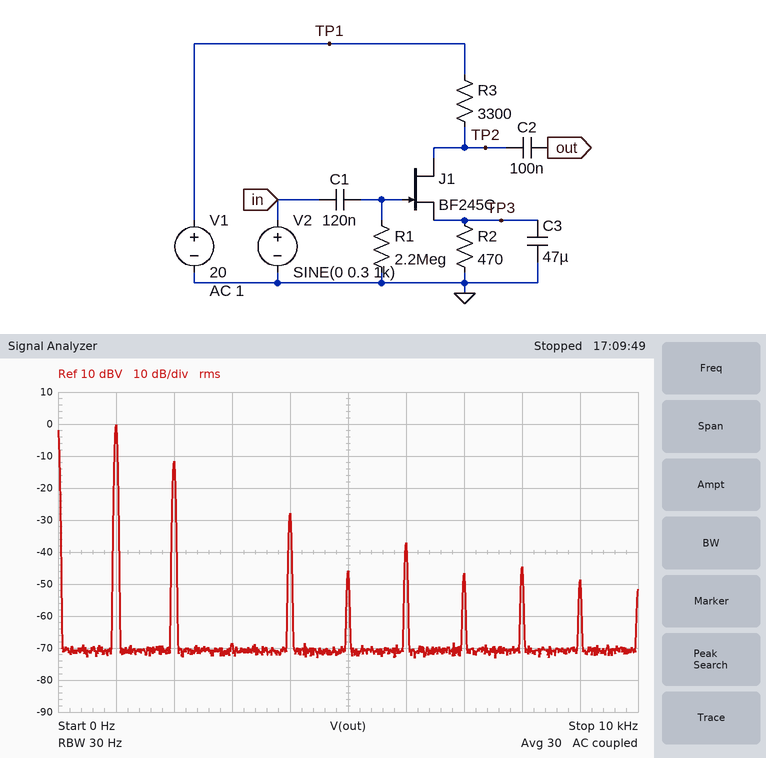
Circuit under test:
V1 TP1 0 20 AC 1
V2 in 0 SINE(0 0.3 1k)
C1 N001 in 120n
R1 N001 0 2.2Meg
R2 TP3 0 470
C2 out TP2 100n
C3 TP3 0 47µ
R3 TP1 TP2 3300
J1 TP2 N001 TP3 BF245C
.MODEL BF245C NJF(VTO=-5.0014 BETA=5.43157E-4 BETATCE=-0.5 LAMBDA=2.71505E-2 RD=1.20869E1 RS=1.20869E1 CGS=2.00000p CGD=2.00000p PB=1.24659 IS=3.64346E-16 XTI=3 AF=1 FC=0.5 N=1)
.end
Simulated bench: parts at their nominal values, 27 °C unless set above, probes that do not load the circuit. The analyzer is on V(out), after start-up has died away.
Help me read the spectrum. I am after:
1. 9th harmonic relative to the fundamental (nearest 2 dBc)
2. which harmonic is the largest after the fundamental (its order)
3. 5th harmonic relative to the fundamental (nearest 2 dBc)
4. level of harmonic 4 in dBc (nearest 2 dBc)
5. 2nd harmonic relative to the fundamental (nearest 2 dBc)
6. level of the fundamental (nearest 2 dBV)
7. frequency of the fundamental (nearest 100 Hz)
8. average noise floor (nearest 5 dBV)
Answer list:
-48 dBc
2
-46 dBc
-28 dBc
-12 dBc
0 dBV
1.0 kHz
-70 dBV
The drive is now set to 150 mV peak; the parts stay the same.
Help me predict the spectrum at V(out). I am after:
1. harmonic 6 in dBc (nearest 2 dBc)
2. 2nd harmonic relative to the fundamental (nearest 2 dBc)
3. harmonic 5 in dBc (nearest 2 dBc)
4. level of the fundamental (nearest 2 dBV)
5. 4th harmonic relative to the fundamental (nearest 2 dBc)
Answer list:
-40 dBc
-14 dBc
-50 dBc
-6 dBV
-30 dBc
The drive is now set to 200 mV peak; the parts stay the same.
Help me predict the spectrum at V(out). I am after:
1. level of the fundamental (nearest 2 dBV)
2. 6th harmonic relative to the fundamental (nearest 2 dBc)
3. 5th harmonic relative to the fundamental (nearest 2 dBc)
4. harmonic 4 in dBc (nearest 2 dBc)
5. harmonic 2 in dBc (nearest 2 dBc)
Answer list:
-4 dBV
-38 dBc
-50 dBc
-30 dBc
-12 dBc
